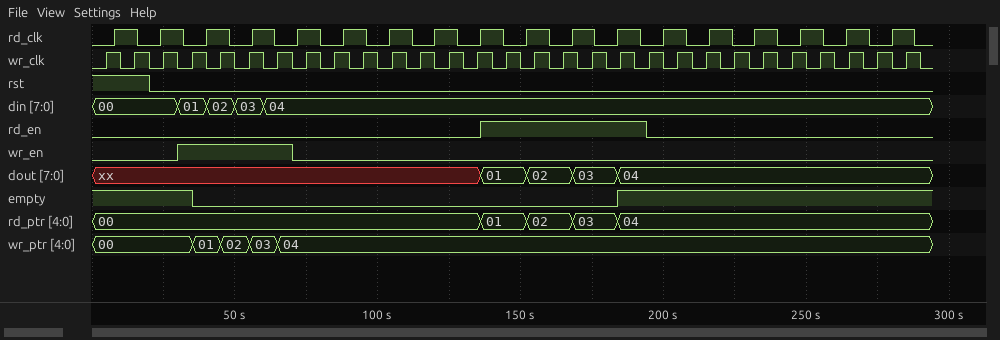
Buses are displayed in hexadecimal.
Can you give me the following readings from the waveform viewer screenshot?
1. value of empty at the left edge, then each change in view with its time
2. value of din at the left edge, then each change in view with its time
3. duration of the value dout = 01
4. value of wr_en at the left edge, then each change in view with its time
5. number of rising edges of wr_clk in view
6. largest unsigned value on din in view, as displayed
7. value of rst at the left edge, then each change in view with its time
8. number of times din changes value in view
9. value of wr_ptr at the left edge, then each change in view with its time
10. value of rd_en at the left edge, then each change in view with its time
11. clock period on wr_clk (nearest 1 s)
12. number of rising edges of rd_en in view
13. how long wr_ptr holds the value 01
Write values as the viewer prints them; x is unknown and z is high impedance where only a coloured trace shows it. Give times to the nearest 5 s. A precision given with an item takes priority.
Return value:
1, 0 at 35 s, 1 at 185 s
00, 01 at 30 s, 02 at 40 s, 03 at 50 s, 04 at 60 s
15 s
0, 1 at 30 s, 0 at 70 s
29
04
1, 0 at 20 s
4
00, 01 at 35 s, 02 at 45 s, 03 at 55 s, 04 at 65 s
0, 1 at 135 s, 0 at 195 s
10 s
1
10 s
